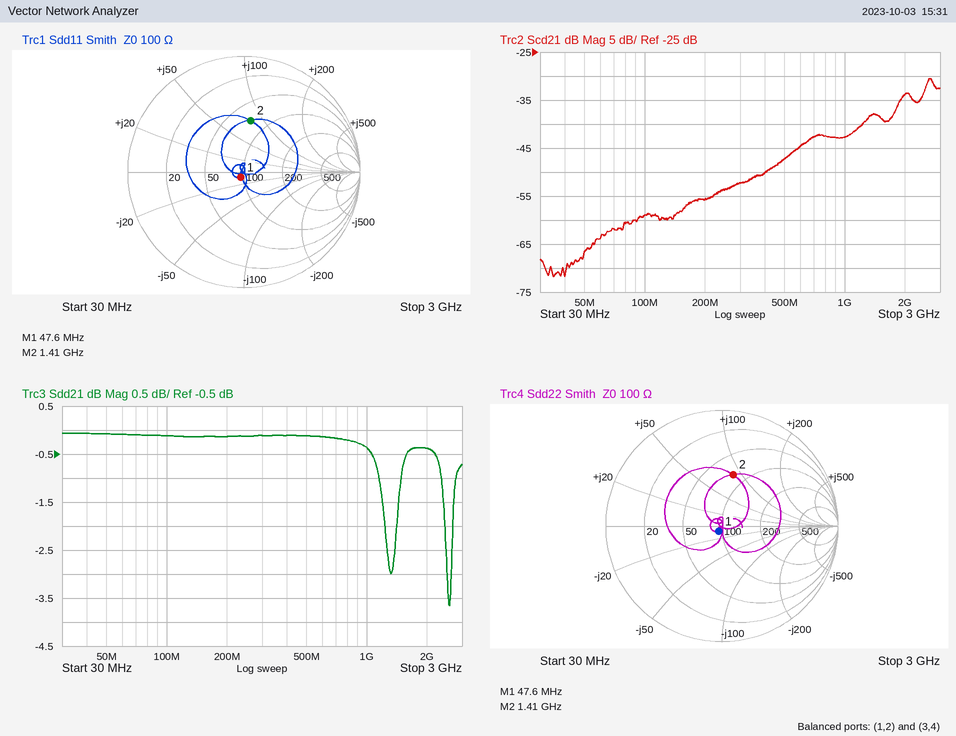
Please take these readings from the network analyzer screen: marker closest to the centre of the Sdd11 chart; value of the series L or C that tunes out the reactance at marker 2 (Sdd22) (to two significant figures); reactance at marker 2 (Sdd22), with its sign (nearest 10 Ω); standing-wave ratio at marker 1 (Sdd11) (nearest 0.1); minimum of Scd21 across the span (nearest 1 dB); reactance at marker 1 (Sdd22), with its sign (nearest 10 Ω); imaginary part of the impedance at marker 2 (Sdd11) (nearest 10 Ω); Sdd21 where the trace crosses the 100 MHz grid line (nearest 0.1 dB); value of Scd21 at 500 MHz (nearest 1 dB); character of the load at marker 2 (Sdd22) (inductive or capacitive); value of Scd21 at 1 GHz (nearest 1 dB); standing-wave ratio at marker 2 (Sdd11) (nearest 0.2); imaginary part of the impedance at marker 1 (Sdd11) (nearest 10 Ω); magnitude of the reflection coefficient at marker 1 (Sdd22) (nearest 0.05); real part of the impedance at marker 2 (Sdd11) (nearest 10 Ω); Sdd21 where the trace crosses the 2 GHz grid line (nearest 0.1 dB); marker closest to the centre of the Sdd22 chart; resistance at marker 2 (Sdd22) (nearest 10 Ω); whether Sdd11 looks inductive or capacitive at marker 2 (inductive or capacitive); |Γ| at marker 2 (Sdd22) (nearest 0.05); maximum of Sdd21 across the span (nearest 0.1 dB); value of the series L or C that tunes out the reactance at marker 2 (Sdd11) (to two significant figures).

marker 1
1.3 pF
+90 Ω
1.1
-72 dB
-10 Ω
+80 Ω
-0.1 dB
-47 dB
inductive
-43 dB
2.6
-10 Ω
0.05
70 Ω
-0.4 dB
marker 1
80 Ω
inductive
0.45
-0.1 dB
1.4 pF
